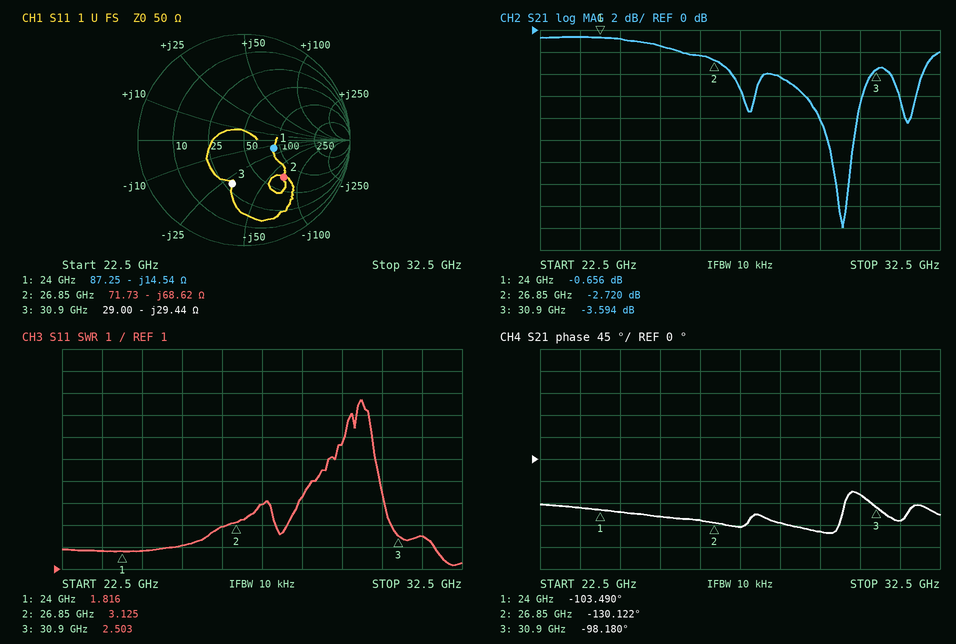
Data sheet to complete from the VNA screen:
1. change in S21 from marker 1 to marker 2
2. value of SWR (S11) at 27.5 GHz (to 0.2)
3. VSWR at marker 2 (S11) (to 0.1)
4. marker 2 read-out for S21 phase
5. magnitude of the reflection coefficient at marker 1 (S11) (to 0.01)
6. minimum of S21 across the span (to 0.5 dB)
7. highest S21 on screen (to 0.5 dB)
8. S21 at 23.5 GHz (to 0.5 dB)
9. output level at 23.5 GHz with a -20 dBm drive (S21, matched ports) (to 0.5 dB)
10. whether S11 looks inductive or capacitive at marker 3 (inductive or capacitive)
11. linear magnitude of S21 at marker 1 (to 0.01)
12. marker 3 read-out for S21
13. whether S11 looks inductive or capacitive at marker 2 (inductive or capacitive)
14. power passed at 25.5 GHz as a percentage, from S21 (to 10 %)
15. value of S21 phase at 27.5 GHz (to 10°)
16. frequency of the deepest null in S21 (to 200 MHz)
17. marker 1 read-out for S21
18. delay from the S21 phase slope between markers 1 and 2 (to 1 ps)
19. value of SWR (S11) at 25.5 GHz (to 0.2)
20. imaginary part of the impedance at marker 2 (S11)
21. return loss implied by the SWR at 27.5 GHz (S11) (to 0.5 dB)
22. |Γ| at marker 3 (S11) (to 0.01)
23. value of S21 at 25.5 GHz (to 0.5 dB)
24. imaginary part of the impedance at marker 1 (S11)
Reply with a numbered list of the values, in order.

1. -2.064 dB
2. 4.0
3. 3.1
4. -130.122°
5. 0.29
6. -18.0 dB
7. -0.5 dB
8. -0.5 dB
9. -20.5 dBm
10. capacitive
11. 0.93
12. -3.594 dB
13. capacitive
14. 70 %
15. -140°
16. 30.0 GHz
17. -0.656 dB
18. 26 ps
19. 2.0
20. -68.62 Ω
21. 4.5 dB
22. 0.43
23. -1.5 dB
24. -14.54 Ω
